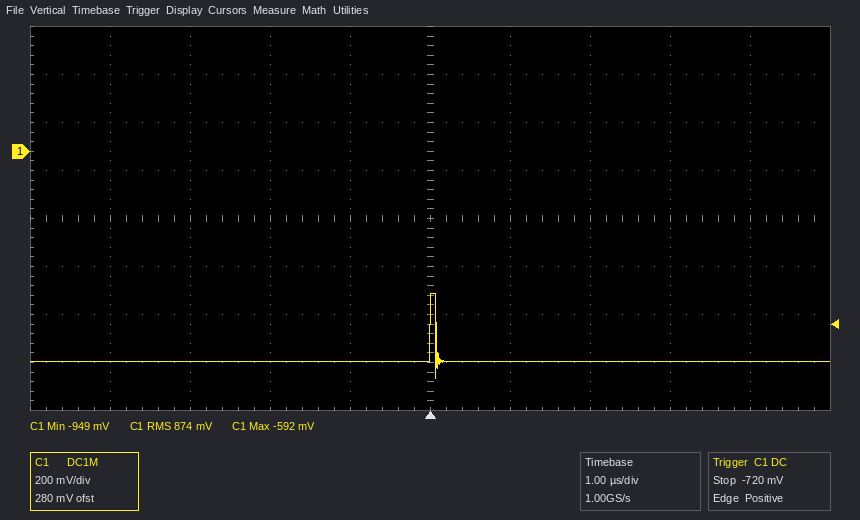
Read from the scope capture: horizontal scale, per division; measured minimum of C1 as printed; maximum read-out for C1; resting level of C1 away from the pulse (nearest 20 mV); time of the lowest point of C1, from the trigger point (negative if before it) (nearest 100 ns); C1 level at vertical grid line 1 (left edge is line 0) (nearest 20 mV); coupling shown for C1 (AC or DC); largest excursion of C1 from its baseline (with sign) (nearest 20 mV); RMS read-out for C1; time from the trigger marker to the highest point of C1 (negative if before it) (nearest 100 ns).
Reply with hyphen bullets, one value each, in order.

- 1 µs
- -949 mV
- -592 mV
- -880 mV
- +100 ns
- -880 mV
- DC
- +280 mV
- 874 mV
- 0.0 µs
